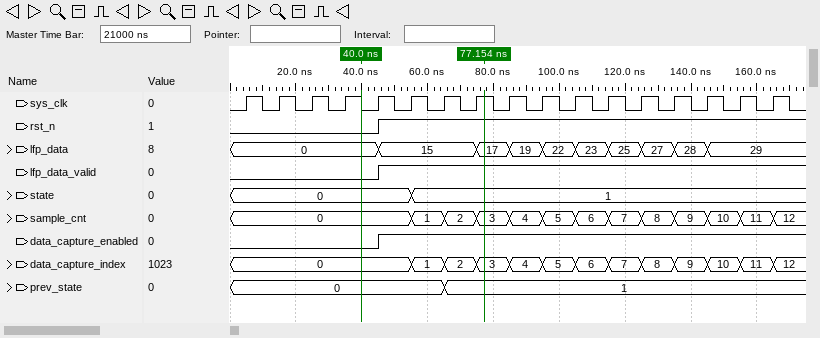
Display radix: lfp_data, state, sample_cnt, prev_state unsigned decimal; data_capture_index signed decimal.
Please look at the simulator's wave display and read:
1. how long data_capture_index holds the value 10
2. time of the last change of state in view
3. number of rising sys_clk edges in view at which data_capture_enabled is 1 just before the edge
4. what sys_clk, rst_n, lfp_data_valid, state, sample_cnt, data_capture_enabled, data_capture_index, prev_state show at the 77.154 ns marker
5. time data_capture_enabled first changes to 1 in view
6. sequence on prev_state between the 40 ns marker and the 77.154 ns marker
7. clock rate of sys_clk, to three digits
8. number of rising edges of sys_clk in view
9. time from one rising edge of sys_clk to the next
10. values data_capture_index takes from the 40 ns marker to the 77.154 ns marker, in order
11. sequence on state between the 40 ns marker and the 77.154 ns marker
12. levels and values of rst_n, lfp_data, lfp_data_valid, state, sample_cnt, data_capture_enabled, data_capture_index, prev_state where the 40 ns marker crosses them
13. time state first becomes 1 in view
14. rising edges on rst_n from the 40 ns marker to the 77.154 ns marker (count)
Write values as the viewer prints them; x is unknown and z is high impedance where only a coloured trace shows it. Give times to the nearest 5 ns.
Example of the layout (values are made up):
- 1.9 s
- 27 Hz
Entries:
- 10 ns
- 55 ns
- 12
- sys_clk=1, rst_n=1, lfp_data_valid=1, state=1, sample_cnt=3, data_capture_enabled=1, data_capture_index=3, prev_state=1
- 45 ns
- 0, 1
- 100 MHz
- 17
- 10 ns
- 0, 1, 2, 3
- 0, 1
- rst_n=0, lfp_data=0, lfp_data_valid=0, state=0, sample_cnt=0, data_capture_enabled=0, data_capture_index=0, prev_state=0
- 55 ns
- 1
